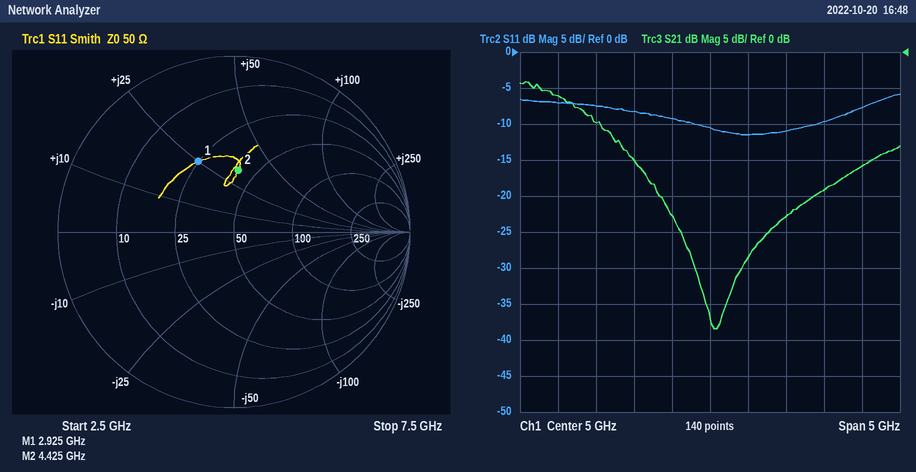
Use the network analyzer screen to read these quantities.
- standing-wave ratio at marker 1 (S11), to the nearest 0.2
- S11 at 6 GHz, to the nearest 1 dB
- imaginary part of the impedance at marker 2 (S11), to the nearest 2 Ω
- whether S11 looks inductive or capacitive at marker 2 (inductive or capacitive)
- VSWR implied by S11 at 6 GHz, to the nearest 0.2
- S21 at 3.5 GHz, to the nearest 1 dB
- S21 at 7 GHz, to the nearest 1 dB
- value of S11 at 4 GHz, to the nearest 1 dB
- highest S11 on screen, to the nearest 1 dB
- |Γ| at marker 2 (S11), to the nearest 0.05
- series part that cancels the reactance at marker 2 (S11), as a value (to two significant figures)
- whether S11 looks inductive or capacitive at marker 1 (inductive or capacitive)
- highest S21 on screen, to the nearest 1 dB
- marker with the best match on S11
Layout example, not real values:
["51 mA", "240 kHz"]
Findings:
["2.6", "-11 dB", "+32 Ω", "inductive", "1.8", "-10 dB", "-16 dB", "-8 dB", "-6 dB", "0.35", "1.1 pF", "inductive", "-4 dB", "marker 2"]
